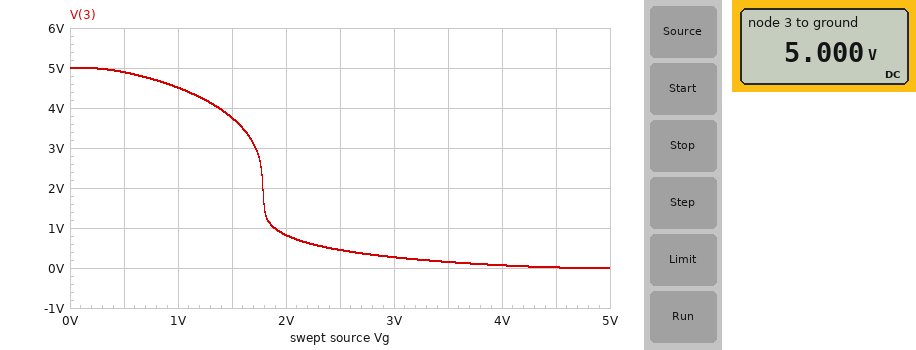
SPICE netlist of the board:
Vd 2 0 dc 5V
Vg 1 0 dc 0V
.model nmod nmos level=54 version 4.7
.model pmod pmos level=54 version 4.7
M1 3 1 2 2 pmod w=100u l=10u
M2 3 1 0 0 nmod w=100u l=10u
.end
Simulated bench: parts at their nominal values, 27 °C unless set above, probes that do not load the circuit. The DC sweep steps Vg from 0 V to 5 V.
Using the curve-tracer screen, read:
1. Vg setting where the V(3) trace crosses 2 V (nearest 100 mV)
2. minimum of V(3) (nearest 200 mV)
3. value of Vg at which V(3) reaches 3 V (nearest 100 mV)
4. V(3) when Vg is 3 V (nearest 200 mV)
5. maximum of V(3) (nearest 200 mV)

1.8 V
0 V
1.7 V
200 mV
5.0 V
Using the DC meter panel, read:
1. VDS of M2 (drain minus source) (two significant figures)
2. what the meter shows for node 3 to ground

5.0 V
5.000 V
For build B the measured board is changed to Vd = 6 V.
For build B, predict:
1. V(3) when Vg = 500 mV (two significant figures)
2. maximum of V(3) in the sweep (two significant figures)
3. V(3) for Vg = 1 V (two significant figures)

5.9 V
6.0 V
5.5 V
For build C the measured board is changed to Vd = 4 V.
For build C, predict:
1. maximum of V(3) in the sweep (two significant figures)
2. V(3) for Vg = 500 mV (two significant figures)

4.0 V
3.9 V
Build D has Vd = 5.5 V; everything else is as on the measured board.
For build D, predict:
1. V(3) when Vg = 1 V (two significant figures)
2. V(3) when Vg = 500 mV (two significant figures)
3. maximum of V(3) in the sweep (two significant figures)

5.0 V
5.4 V
5.5 V
